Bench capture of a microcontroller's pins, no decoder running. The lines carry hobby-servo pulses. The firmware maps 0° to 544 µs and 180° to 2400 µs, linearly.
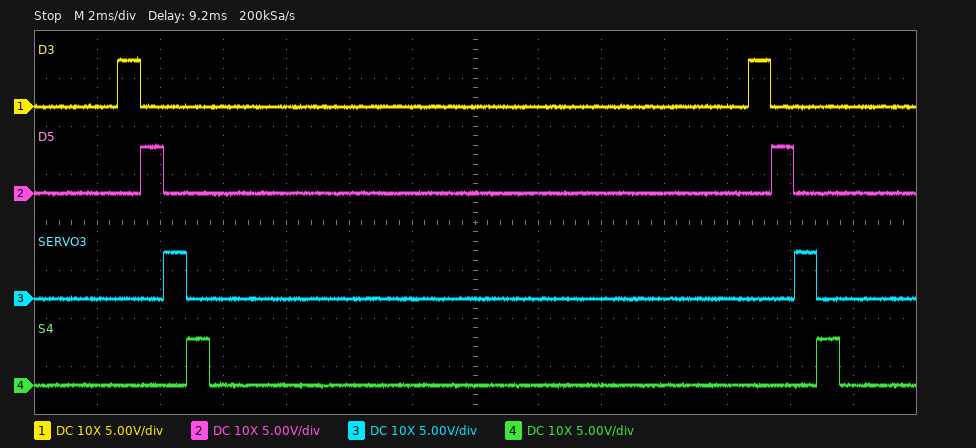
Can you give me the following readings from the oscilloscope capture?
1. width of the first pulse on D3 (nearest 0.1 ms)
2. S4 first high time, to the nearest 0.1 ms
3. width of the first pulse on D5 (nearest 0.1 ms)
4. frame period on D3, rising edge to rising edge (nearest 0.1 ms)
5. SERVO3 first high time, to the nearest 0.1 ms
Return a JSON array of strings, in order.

["0.7 ms", "0.7 ms", "0.7 ms", "20.0 ms", "0.7 ms"]
